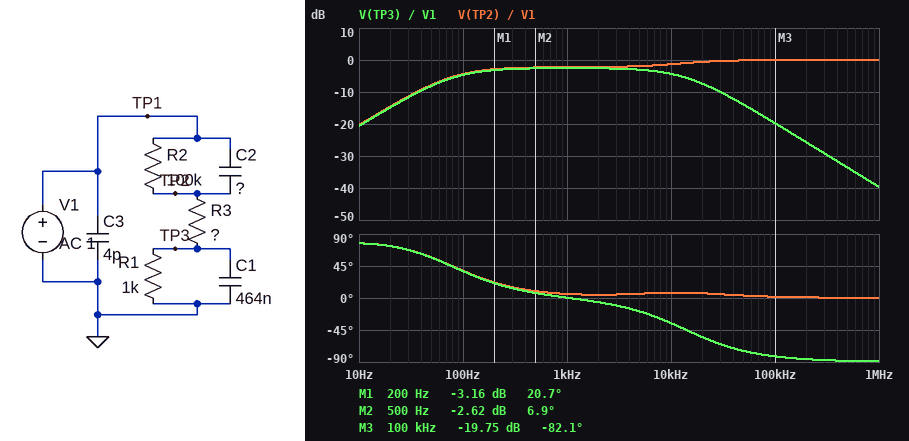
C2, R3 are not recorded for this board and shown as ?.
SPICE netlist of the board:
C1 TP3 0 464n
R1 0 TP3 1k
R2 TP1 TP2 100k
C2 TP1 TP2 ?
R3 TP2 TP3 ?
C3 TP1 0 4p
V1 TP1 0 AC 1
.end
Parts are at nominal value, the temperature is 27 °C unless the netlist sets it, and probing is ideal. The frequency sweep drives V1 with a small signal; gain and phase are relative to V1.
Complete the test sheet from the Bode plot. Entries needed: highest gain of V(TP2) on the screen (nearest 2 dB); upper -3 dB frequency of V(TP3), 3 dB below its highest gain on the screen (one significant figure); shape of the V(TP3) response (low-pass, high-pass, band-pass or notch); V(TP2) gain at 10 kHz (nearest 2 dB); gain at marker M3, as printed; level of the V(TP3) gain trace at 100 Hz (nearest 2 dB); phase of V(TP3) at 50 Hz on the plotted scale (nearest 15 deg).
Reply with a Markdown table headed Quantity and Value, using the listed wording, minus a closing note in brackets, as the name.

| Quantity | Value |
|---|---|
| highest gain of V(TP2) on the screen | 0 dB |
| upper -3 dB frequency of V(TP3), 3 dB below its highest gain on the screen | 10 kHz |
| shape of the V(TP3) response | band-pass |
| V(TP2) gain at 10 kHz | -2 dB |
| gain at marker M3, as printed | -19.75 dB |
| level of the V(TP3) gain trace at 100 Hz | -4 dB |
| phase of V(TP3) at 50 Hz on the plotted scale | 60 deg |
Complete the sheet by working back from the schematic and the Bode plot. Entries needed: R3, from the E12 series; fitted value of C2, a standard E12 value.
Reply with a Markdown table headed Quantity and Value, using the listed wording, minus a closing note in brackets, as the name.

| Quantity | Value |
|---|---|
| R3, from the E12 series | 33 Ω |
| fitted value of C2, a standard E12 value | 1.5 µF |
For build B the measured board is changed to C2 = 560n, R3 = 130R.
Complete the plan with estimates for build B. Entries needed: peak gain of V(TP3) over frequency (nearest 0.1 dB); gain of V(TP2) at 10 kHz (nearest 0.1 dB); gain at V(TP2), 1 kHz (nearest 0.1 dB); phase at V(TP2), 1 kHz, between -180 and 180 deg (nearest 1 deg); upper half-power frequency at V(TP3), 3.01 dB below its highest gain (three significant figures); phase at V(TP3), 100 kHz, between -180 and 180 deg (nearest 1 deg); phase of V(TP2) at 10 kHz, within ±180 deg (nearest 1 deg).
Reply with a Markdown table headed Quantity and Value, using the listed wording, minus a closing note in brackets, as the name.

| Quantity | Value |
|---|---|
| peak gain of V(TP3) over frequency | -5.8 dB |
| gain of V(TP2) at 10 kHz | -0.6 dB |
| gain at V(TP2), 1 kHz | -4.3 dB |
| phase at V(TP2), 1 kHz, between -180 and 180 deg | 16 deg |
| upper half-power frequency at V(TP3), 3.01 dB below its highest gain | 5.31 kHz |
| phase at V(TP3), 100 kHz, between -180 and 180 deg | -87 deg |
| phase of V(TP2) at 10 kHz, within ±180 deg | 11 deg |
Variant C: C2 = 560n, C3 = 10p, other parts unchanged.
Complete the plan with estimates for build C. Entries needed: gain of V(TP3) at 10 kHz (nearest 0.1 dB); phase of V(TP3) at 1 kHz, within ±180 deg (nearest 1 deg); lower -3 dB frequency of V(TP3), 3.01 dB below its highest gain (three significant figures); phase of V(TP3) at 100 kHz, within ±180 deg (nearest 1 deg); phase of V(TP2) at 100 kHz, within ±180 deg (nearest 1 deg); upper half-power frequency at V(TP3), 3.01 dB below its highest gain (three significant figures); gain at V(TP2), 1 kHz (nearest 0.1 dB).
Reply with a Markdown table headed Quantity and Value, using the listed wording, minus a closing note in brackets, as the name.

| Quantity | Value |
|---|---|
| gain of V(TP3) at 10 kHz | -6.4 dB |
| phase of V(TP3) at 1 kHz, within ±180 deg | 6 deg |
| lower -3 dB frequency of V(TP3), 3.01 dB below its highest gain | 153 Hz |
| phase of V(TP3) at 100 kHz, within ±180 deg | -79 deg |
| phase of V(TP2) at 100 kHz, within ±180 deg | 5 deg |
| upper half-power frequency at V(TP3), 3.01 dB below its highest gain | 19.5 kHz |
| gain at V(TP2), 1 kHz | -5.1 dB |
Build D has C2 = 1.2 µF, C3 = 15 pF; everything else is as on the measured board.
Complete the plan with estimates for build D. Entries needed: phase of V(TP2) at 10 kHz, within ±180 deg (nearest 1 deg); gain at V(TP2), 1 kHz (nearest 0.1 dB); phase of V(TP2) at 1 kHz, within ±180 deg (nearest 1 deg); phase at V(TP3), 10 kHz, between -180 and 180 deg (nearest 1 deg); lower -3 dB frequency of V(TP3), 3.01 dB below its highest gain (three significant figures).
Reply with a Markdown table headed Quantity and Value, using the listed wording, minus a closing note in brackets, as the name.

| Quantity | Value |
|---|---|
| phase of V(TP2) at 10 kHz, within ±180 deg | 9 deg |
| gain at V(TP2), 1 kHz | -2.7 dB |
| phase of V(TP2) at 1 kHz, within ±180 deg | 7 deg |
| phase at V(TP3), 10 kHz, between -180 and 180 deg | -34 deg |
| lower -3 dB frequency of V(TP3), 3.01 dB below its highest gain | 93.8 Hz |
